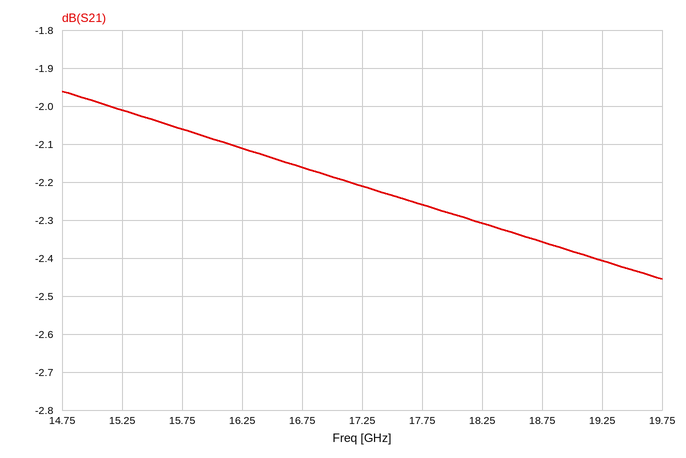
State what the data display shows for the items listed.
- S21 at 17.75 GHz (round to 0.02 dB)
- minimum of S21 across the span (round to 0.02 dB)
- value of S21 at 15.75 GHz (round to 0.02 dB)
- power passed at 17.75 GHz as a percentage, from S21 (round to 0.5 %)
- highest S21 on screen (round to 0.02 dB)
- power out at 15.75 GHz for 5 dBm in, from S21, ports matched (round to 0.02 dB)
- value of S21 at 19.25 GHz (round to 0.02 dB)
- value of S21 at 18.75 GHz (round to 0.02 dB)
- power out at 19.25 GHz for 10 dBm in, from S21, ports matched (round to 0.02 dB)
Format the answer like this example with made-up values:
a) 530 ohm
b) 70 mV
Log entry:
a) -2.26 dB
b) -2.46 dB
c) -2.06 dB
d) 59.5 %
e) -1.96 dB
f) 2.94 dBm
g) -2.40 dB
h) -2.36 dB
i) 7.60 dBm
